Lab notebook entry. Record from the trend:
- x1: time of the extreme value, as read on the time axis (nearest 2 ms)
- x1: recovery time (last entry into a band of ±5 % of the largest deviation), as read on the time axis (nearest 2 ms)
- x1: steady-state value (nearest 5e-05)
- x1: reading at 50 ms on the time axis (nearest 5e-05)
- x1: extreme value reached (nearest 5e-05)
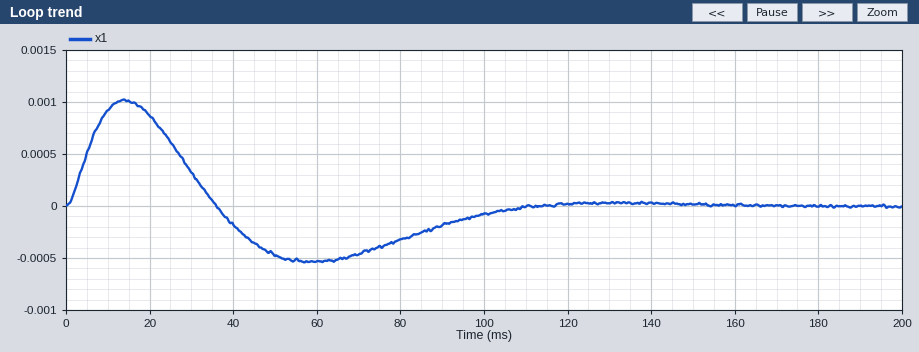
14 ms
104 ms
0.00000
-0.00045
0.00100
